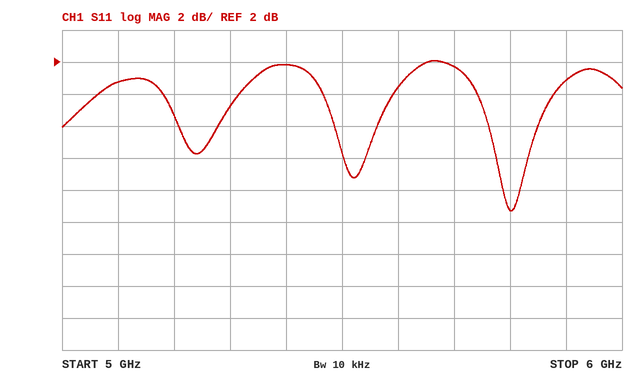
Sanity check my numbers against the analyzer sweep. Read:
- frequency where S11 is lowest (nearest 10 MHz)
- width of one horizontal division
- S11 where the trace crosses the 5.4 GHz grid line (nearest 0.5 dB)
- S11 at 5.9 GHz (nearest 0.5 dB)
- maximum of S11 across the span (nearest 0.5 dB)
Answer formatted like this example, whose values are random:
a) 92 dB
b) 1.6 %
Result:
a) 5.80 GHz
b) 100 MHz
c) 2.0 dB
d) 1.0 dB
e) 2.0 dB
